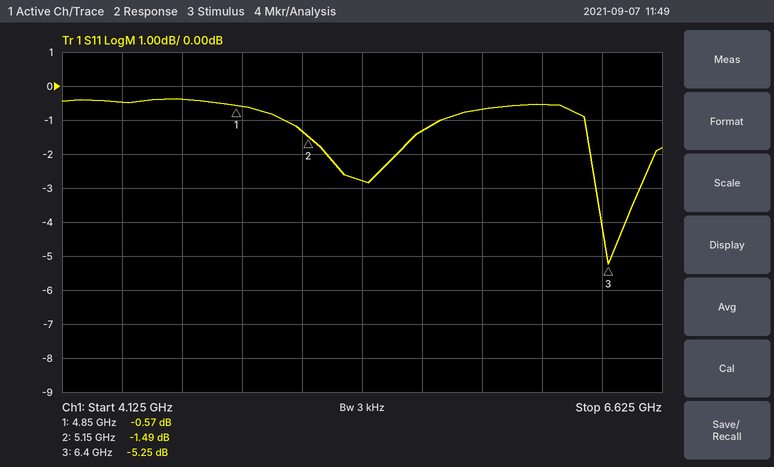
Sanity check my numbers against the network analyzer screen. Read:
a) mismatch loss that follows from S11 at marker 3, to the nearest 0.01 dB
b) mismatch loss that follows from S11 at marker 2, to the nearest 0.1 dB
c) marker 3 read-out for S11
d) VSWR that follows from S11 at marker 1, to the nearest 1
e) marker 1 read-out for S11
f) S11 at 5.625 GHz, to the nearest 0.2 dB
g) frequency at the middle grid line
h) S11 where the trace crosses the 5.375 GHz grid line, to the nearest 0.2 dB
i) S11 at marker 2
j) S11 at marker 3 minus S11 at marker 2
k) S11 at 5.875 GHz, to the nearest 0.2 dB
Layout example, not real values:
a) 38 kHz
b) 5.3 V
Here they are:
a) 1.54 dB
b) 5.4 dB
c) -5.25 dB
d) 30
e) -0.57 dB
f) -1.4 dB
g) 5.375 GHz
h) -2.8 dB
i) -1.49 dB
j) -3.76 dB
k) -0.6 dB
